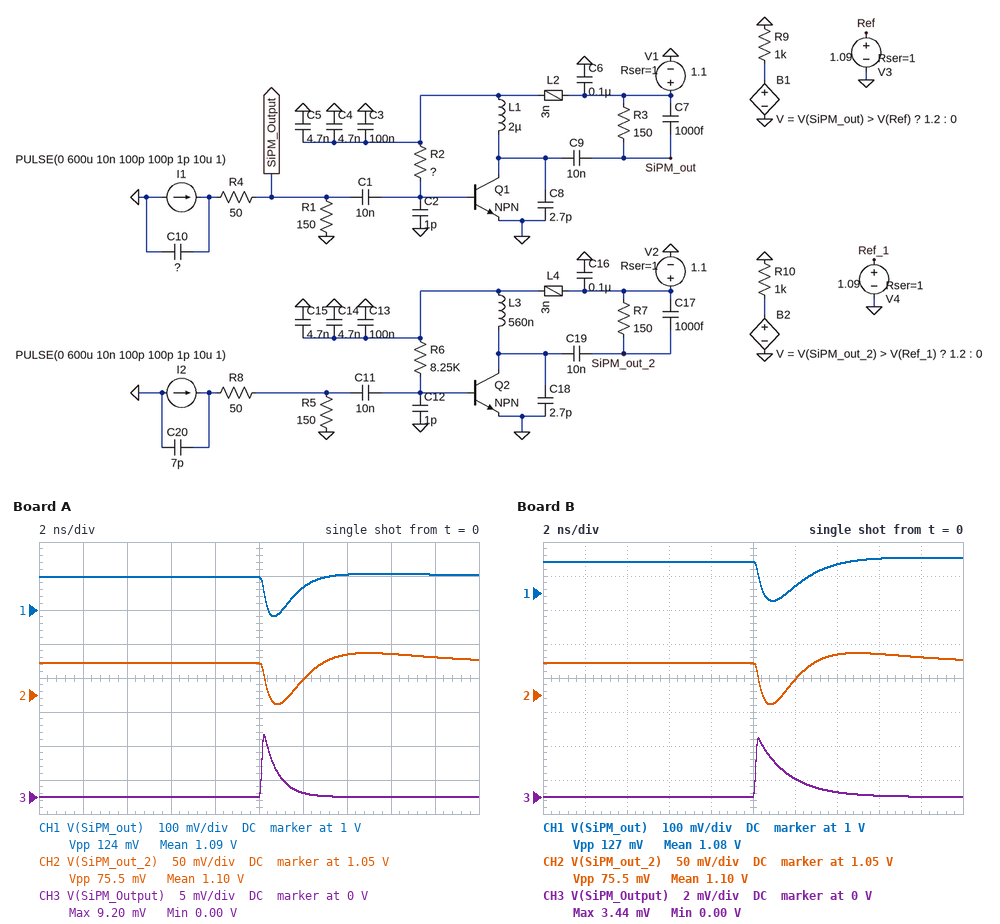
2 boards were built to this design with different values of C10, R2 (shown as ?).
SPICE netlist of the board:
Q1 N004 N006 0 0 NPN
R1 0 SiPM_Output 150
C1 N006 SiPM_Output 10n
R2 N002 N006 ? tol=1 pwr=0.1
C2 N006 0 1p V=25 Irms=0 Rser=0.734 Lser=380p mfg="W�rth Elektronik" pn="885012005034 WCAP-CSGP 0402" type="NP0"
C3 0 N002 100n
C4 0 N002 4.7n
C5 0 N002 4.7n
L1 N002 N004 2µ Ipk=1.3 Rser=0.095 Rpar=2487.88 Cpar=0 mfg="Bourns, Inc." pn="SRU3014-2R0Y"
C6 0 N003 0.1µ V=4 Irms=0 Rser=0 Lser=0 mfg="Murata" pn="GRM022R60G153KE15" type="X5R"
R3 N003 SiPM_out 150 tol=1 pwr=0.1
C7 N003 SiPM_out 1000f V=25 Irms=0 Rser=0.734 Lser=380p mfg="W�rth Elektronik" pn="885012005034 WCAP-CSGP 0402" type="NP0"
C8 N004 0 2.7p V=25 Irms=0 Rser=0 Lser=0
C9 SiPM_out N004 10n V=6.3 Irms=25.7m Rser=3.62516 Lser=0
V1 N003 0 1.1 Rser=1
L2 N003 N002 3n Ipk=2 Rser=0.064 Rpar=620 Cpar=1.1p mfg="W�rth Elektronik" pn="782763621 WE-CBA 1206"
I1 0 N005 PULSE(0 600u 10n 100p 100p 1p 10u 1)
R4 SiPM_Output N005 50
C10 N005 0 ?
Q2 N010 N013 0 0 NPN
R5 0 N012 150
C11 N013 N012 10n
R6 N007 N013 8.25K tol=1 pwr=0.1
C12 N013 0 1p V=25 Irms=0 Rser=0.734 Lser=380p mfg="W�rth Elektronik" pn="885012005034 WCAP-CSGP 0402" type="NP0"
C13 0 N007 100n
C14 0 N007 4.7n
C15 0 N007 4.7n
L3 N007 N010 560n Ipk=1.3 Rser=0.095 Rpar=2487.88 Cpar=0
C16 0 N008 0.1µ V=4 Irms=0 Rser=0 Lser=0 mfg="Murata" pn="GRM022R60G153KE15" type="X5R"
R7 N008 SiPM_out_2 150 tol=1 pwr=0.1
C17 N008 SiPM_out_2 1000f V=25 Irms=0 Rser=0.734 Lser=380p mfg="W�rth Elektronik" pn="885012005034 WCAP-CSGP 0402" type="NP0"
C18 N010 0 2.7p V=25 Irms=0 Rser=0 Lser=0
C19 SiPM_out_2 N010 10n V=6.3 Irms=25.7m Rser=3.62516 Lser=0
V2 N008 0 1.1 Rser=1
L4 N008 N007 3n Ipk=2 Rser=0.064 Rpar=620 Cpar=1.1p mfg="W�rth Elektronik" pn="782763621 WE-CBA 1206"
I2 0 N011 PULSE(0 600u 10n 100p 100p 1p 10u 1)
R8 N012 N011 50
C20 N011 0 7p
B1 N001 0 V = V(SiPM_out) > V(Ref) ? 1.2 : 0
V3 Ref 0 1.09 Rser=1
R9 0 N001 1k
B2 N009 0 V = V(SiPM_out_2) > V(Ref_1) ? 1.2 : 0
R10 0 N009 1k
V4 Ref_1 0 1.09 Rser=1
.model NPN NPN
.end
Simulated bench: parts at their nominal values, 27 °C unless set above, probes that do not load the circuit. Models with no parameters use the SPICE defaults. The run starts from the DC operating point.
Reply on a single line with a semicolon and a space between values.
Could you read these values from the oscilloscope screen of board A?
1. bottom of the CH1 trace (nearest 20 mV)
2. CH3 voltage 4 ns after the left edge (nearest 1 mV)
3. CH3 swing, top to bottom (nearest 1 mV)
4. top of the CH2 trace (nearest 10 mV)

980 mV; 0 V; 9 mV; 1.11 V
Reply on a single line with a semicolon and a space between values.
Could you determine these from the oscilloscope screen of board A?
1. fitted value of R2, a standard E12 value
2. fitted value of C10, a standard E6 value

6.8 kΩ; 3.3 pF
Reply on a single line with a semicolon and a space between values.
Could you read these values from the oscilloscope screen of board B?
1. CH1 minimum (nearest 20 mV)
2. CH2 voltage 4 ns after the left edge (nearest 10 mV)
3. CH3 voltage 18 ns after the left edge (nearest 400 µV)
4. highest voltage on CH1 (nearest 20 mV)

980 mV; 1.10 V; 0 V; 1.10 V
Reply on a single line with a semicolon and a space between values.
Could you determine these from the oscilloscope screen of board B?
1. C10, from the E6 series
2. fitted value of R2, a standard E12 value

10 pF; 2.7 kΩ
